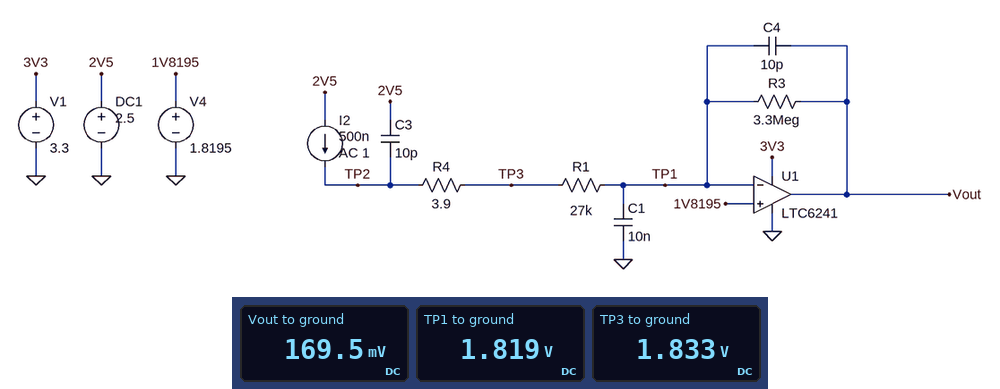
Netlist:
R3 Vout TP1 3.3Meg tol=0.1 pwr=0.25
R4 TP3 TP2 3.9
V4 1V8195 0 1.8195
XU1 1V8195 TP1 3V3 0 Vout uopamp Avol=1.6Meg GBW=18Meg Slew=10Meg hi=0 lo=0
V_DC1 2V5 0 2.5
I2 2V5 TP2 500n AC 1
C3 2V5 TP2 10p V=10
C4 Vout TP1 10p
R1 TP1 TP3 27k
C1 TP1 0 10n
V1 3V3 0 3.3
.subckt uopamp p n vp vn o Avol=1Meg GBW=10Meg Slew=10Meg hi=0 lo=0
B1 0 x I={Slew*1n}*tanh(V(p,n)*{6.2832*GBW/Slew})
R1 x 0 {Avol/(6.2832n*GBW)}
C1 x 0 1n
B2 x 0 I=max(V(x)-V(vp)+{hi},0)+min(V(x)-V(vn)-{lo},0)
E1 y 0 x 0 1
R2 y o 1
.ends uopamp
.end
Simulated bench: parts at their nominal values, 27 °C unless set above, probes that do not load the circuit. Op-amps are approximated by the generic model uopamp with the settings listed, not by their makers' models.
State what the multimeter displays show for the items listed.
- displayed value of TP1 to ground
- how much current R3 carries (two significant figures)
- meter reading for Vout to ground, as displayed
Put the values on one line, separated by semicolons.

1.819 V; 500 nA; 169.5 mV
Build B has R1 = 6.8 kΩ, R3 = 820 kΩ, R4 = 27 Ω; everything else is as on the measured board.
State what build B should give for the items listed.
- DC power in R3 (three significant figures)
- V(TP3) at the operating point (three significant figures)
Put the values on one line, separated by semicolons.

205 nW; 1.82 V
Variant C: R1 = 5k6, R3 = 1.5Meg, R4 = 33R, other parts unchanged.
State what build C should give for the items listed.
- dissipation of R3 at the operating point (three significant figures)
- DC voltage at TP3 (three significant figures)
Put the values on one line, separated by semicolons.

375 nW; 1.82 V
